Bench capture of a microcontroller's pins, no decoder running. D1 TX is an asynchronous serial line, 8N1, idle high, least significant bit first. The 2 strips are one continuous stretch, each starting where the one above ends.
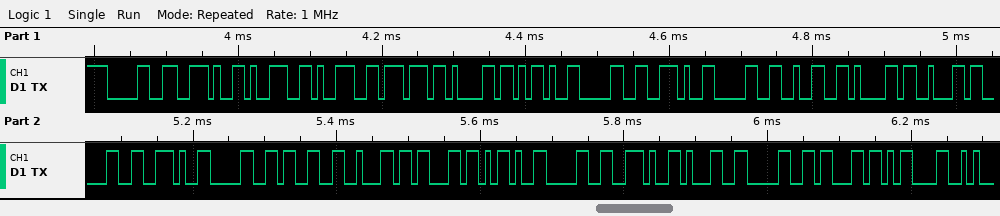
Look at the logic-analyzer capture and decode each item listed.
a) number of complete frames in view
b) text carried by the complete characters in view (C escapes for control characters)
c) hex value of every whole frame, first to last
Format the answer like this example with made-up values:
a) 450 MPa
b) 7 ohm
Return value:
a) 26
b) "0.99wa-0.02ab0.03bc-0.10c\r"
c) 30 2E 39 39 77 61 2D 30 2E 30 32 61 62 30 2E 30 33 62 63 2D 30 2E 31 30 63 0D
